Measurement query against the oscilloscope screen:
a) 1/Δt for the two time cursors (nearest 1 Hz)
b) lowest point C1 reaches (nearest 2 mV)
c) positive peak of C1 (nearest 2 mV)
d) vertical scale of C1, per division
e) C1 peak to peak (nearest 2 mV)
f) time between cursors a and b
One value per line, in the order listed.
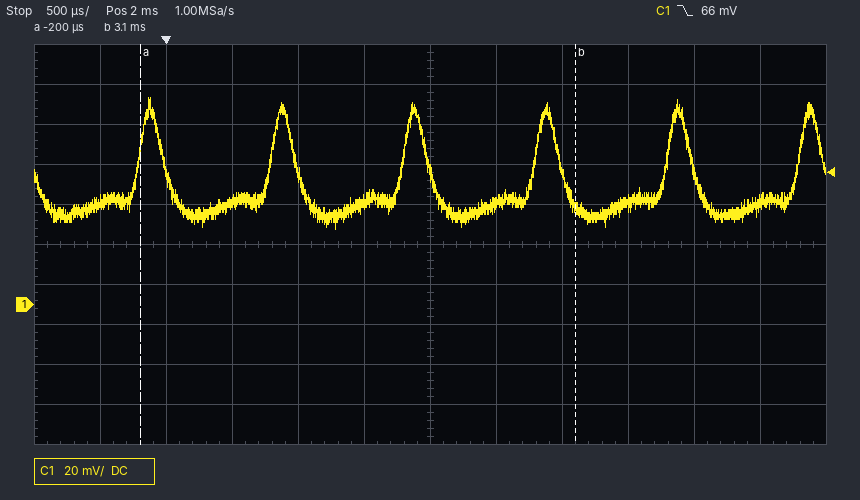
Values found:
303 Hz
38 mV
104 mV
20 mV
66 mV
3.30 ms
